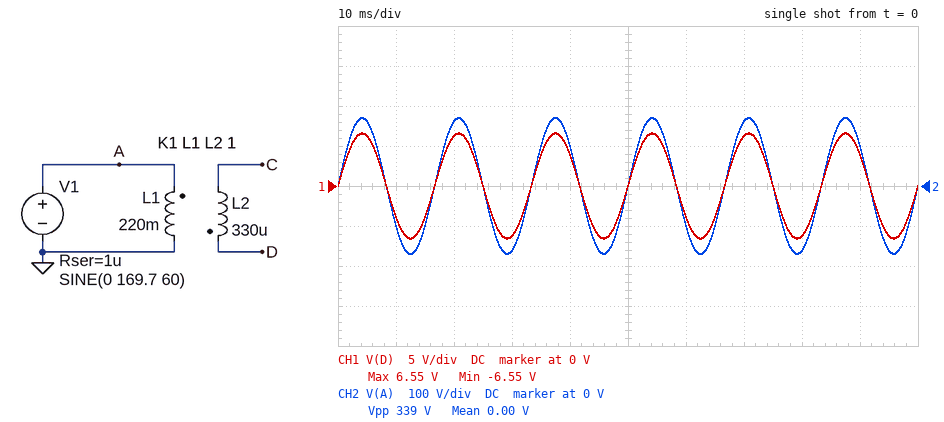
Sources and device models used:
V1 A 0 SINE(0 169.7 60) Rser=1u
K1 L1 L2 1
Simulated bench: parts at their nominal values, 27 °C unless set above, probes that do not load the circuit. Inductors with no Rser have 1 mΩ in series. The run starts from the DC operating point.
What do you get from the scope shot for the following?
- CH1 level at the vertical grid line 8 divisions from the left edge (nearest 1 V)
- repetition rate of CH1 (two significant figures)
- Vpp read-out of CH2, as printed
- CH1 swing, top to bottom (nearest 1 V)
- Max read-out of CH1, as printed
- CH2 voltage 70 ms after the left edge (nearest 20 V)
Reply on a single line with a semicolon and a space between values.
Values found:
-6 V; 60 Hz; 339 V; 13 V; 6.55 V; 160 V
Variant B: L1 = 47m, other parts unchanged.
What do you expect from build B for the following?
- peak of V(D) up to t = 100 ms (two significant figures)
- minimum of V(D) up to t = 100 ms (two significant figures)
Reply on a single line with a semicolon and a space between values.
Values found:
14 V; -14 V
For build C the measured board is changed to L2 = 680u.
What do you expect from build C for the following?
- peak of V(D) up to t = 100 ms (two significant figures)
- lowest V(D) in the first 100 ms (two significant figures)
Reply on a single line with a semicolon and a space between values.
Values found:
9.4 V; -9.4 V
